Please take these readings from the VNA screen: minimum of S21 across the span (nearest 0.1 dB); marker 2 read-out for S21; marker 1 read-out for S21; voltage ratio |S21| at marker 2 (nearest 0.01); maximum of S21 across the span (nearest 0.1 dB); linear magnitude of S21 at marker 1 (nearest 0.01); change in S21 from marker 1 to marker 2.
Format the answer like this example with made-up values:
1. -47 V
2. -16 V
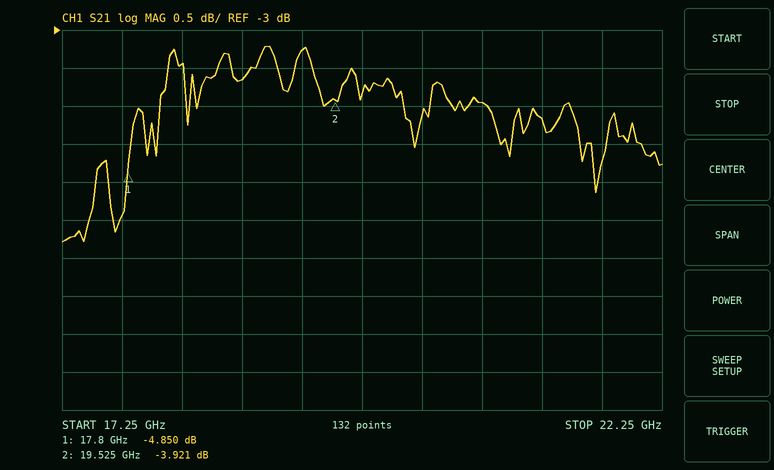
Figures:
1. -5.8 dB
2. -3.921 dB
3. -4.850 dB
4. 0.64
5. -3.2 dB
6. 0.57
7. 0.929 dB
